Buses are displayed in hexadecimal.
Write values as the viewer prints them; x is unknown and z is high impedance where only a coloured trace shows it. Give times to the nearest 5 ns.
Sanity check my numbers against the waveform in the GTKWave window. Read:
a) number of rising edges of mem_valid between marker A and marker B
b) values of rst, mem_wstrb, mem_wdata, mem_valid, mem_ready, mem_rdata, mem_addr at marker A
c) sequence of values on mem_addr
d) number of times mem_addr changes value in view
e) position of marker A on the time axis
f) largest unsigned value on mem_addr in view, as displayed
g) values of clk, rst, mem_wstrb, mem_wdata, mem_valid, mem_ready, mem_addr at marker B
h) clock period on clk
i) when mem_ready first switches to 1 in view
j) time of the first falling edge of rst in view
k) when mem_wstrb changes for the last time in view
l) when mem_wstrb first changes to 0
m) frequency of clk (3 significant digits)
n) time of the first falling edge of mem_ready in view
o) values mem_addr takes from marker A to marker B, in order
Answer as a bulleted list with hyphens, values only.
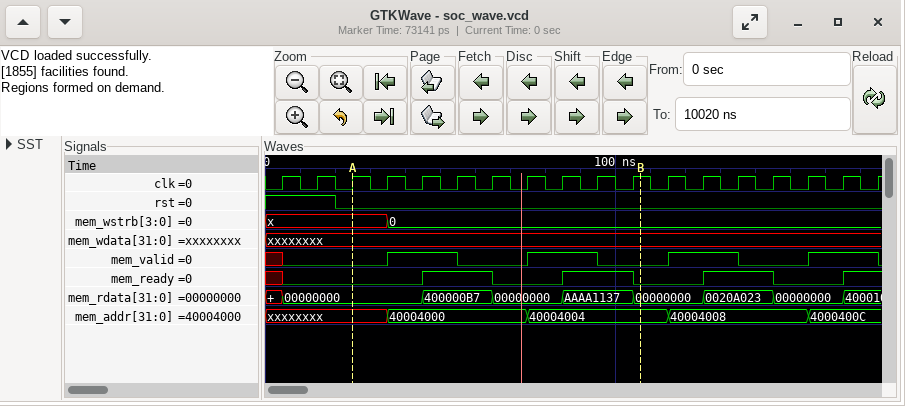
- 2
- rst=0, mem_wstrb=x, mem_wdata=xxxxxxxx, mem_valid=0, mem_ready=0, mem_rdata=00000000, mem_addr=xxxxxxxx
- xxxxxxxx, 40004000, 40004004, 40004008, 4000400C
- 4
- 25 ns
- 4000400C
- clk=1, rst=0, mem_wstrb=0, mem_wdata=xxxxxxxx, mem_valid=0, mem_ready=0, mem_addr=40004004
- 10 ns
- 45 ns
- 20 ns
- 35 ns
- 35 ns
- 100 MHz
- 65 ns
- xxxxxxxx, 40004000, 40004004
